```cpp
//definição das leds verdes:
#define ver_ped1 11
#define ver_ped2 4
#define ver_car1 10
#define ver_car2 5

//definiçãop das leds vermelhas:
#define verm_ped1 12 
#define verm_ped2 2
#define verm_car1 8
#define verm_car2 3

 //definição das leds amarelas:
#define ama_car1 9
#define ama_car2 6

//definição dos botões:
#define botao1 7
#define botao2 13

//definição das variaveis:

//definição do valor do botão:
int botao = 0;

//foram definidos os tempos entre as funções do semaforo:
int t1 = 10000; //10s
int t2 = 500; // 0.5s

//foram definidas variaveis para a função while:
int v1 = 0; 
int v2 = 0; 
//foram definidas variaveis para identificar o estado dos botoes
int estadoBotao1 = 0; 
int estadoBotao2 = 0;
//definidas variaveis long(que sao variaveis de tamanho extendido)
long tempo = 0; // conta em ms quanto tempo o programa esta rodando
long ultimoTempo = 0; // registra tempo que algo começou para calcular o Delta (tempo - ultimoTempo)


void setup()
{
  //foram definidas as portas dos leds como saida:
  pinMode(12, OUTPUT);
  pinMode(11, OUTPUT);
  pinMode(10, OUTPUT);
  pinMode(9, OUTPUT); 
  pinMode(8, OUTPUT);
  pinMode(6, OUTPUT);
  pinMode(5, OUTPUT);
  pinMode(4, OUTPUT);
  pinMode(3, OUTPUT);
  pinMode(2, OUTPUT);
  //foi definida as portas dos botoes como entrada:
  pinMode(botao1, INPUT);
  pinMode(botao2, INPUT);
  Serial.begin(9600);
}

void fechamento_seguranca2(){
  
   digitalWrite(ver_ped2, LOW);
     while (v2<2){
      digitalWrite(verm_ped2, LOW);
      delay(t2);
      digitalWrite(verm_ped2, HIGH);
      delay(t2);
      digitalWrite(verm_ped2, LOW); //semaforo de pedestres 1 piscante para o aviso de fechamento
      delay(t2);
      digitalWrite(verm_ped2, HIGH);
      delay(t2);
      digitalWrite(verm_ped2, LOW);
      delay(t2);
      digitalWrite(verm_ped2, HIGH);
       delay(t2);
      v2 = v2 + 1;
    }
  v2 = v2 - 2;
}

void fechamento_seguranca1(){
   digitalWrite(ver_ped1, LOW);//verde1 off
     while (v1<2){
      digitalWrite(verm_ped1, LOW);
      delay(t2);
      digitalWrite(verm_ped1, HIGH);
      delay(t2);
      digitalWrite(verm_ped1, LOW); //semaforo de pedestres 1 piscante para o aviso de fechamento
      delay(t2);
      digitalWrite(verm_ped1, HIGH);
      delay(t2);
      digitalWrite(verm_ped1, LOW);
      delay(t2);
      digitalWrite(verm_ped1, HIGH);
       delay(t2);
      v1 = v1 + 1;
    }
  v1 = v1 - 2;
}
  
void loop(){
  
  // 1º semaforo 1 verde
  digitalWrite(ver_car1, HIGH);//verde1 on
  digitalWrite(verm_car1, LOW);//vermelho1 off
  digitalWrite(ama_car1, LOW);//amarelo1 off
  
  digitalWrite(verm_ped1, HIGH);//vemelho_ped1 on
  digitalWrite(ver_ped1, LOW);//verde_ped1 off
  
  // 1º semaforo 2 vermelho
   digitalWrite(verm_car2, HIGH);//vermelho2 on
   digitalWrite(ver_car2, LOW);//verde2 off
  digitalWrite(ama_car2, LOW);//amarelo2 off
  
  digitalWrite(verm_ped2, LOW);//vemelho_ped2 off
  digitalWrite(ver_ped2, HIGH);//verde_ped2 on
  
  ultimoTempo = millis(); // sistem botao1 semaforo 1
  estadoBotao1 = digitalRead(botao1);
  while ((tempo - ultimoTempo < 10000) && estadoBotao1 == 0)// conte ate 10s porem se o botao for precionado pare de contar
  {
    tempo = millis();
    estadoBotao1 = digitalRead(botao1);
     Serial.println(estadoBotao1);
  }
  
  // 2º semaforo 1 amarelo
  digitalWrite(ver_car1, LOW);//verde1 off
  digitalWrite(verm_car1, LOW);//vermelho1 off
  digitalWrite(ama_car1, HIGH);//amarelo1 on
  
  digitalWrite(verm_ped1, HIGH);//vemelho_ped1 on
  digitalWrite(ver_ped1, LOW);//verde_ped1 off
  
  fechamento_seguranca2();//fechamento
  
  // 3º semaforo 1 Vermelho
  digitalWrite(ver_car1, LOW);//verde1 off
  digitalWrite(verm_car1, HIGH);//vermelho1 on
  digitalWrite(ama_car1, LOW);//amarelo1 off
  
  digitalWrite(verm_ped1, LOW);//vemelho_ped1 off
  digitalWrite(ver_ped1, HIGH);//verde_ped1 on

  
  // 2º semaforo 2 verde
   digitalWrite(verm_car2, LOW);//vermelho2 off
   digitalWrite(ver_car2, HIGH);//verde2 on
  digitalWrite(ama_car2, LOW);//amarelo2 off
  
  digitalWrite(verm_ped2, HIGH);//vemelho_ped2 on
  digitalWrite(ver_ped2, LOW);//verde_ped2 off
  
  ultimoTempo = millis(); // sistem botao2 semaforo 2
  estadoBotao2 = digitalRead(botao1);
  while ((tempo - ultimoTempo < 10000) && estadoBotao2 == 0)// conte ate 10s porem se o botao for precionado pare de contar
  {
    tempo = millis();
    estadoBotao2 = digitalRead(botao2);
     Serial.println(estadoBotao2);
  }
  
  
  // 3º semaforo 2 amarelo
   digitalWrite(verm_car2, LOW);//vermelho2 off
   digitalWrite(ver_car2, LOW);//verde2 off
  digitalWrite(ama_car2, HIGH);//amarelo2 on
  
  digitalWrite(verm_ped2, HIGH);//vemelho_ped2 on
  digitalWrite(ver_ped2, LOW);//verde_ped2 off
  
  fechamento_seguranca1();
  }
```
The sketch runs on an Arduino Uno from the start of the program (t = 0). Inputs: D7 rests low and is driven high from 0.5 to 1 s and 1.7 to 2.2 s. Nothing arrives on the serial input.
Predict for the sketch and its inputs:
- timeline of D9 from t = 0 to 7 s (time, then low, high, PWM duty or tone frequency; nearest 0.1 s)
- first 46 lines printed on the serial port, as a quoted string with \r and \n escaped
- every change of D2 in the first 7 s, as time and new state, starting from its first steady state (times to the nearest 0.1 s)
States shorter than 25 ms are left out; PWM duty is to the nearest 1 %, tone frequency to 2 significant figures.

0 s low; 0.5 s high; 6.5 s low
"0\r\n0\r\n0\r\n0\r\n0\r\n0\r\n0\r\n0\r\n0\r\n0\r\n0\r\n0\r\n0\r\n0\r\n0\r\n0\r\n0\r\n0\r\n0\r\n0\r\n0\r\n0\r\n0\r\n0\r\n0\r\n0\r\n0\r\n0\r\n0\r\n0\r\n0\r\n0\r\n0\r\n0\r\n0\r\n0\r\n0\r\n0\r\n0\r\n0\r\n0\r\n0\r\n0\r\n0\r\n0\r\n0\r\n"
0 s low; 1 s high; 1.5 s low; 2 s high; 2.5 s low; 3 s high; 3.5 s low; 4 s high; 4.5 s low; 5 s high; 5.5 s low; 6 s high
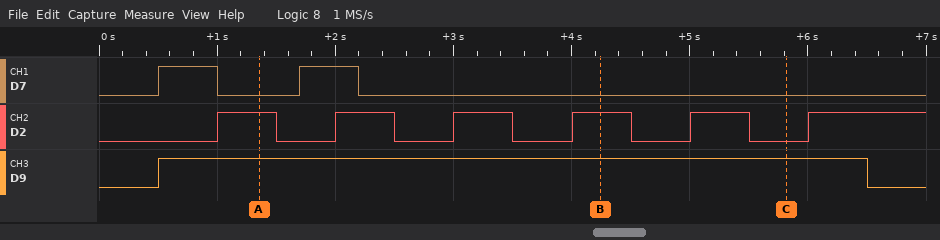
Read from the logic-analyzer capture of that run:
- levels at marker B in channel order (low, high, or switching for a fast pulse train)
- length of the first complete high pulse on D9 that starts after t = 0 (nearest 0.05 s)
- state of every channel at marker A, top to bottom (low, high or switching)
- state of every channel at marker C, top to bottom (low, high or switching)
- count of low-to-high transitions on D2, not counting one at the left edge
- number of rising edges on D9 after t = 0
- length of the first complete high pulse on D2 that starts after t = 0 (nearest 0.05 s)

D7 low, D2 high, D9 high
6.00 s
D7 low, D2 high, D9 high
D7 low, D2 low, D9 high
6
1
0.50 s
